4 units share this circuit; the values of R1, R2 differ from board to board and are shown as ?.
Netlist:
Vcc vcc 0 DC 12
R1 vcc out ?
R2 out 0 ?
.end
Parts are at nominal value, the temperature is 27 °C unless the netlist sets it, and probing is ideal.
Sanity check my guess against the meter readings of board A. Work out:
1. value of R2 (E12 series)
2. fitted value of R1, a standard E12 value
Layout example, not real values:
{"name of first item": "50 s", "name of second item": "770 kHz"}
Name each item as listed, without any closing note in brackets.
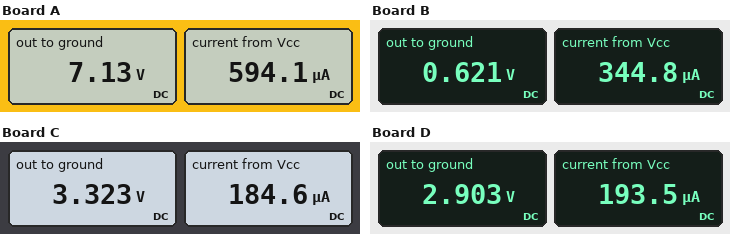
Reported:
{"value of R2": "12 kΩ", "fitted value of R1, a standard E12 value": "8.2 kΩ"}
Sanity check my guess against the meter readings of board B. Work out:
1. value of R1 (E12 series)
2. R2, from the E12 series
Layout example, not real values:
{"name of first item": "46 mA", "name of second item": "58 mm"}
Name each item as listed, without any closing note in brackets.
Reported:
{"value of R1": "33 kΩ", "R2, from the E12 series": "1.8 kΩ"}
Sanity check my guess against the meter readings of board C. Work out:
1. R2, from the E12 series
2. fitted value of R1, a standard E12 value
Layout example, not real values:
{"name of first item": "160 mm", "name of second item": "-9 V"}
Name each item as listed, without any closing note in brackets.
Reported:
{"R2, from the E12 series": "18 kΩ", "fitted value of R1, a standard E12 value": "47 kΩ"}
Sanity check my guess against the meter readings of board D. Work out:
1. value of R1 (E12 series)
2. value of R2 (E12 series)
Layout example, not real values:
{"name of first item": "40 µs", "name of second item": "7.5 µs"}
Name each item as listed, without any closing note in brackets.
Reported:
{"value of R1": "47 kΩ", "value of R2": "15 kΩ"}
